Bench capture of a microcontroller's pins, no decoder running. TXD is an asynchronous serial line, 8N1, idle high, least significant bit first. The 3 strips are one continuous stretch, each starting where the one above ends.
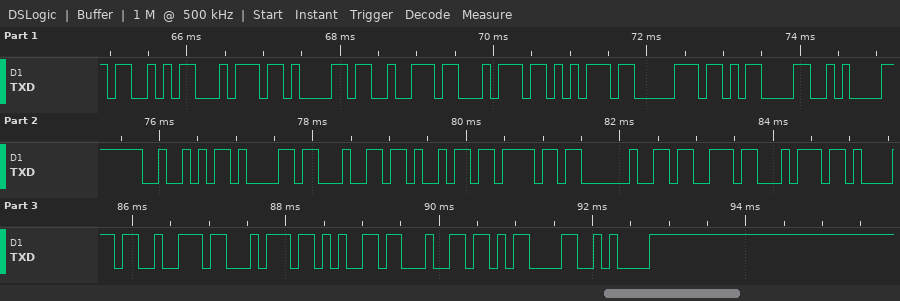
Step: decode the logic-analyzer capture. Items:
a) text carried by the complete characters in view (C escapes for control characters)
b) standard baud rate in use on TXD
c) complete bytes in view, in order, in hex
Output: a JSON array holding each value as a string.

["\"Startup\\r\\nRadio started\\r\\n\"", "9600 baud", "0x53 0x74 0x61 0x72 0x74 0x75 0x70 0x0D 0x0A 0x52 0x61 0x64 0x69 0x6F 0x20 0x73 0x74 0x61 0x72 0x74 0x65 0x64 0x0D 0x0A"]
